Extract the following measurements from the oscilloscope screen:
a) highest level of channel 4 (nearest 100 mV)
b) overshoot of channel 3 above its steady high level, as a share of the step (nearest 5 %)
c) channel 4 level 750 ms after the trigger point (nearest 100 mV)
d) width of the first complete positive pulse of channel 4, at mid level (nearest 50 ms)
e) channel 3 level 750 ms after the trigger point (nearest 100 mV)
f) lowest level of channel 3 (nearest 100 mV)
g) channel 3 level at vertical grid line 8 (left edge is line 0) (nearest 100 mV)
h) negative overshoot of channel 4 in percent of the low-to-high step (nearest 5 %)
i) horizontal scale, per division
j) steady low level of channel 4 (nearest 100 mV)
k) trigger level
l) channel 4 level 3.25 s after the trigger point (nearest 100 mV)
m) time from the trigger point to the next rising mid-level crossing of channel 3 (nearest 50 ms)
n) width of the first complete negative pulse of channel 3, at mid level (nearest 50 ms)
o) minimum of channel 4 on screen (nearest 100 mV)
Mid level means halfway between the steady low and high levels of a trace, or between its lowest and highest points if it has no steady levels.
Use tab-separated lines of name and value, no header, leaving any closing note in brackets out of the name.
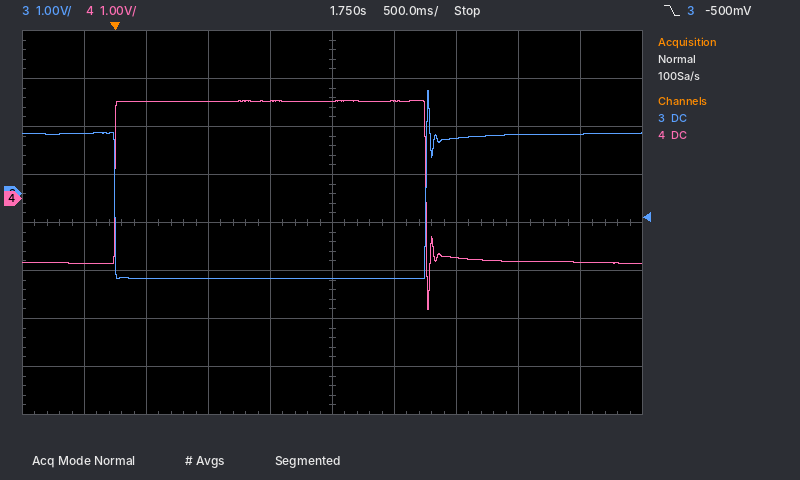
highest level of channel 4	2.0 V
overshoot of channel 3 above its steady high level, as a share of the step	30 %
channel 4 level 750 ms after the trigger point	2.0 V
width of the first complete positive pulse of channel 4, at mid level	2.50 s
channel 3 level 750 ms after the trigger point	-1.8 V
lowest level of channel 3	-1.8 V
channel 3 level at vertical grid line 8 (left edge is line 0)	1.2 V
negative overshoot of channel 4 in percent of the low-to-high step	30 %
horizontal scale, per division	500 ms
steady low level of channel 4	-1.3 V
trigger level	-500 mV
channel 4 level 3.25 s after the trigger point	-1.3 V
time from the trigger point to the next rising mid-level crossing of channel 3	2.50 s
width of the first complete negative pulse of channel 3, at mid level	2.50 s
minimum of channel 4 on screen	-2.3 V
